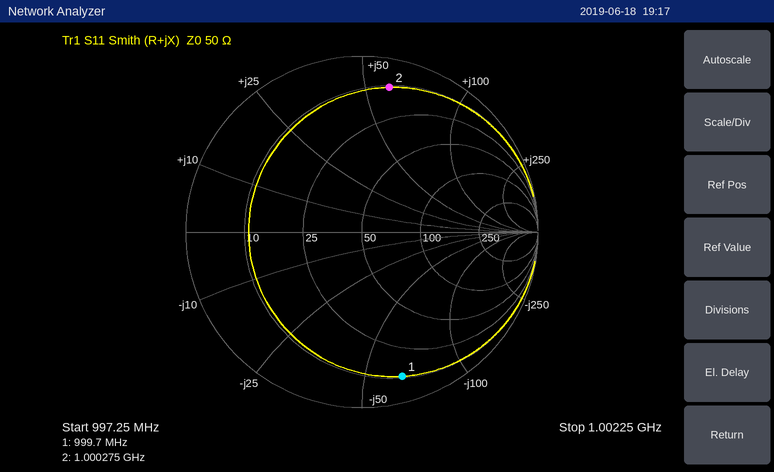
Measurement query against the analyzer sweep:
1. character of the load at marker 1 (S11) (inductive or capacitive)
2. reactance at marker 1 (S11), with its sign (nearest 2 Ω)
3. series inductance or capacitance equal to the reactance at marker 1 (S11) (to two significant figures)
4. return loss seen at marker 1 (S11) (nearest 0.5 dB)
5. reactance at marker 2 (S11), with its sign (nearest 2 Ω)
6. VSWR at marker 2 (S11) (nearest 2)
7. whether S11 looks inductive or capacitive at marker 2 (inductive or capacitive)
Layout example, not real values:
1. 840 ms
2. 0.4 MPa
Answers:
1. capacitive
2. -64 Ω
3. 2.5 pF
4. 1.5 dB
5. +60 Ω
6. 12
7. inductive
